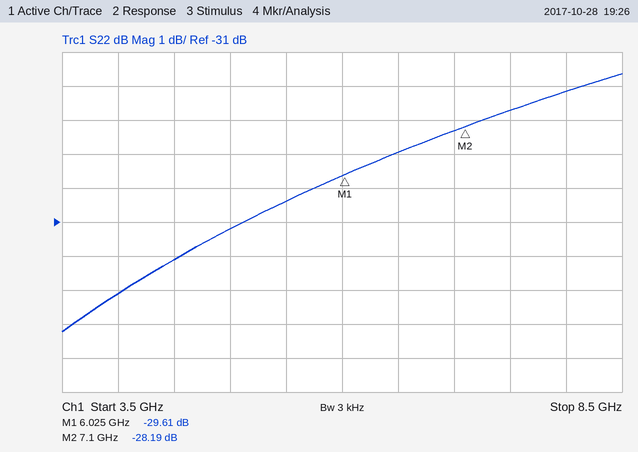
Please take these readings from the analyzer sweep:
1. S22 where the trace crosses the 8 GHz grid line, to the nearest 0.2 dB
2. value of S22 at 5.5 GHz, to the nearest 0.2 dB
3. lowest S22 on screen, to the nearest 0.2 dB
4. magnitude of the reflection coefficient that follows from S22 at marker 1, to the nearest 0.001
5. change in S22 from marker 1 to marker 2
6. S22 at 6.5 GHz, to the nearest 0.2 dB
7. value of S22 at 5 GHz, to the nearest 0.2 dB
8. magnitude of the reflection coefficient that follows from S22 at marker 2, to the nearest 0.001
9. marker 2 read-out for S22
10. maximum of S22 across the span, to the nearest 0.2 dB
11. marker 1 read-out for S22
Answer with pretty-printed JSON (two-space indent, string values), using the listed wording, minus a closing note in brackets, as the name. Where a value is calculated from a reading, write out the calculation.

{
  "S22 where the trace crosses the 8 GHz grid line, to the nearest 0.2 dB": "-27.2 dB",
  "value of S22 at 5.5 GHz, to the nearest 0.2 dB": "-30.4 dB",
  "lowest S22 on screen, to the nearest 0.2 dB": "-34.2 dB",
  "magnitude of the reflection coefficient that follows from S22 at marker 1, to the nearest 0.001": "10^(-29.61/20) ≈ 0.033",
  "change in S22 from marker 1 to marker 2": "-28.19 − (-29.61) = 1.42 dB",
  "S22 at 6.5 GHz, to the nearest 0.2 dB": "-29.0 dB",
  "value of S22 at 5 GHz, to the nearest 0.2 dB": "-31.2 dB",
  "magnitude of the reflection coefficient that follows from S22 at marker 2, to the nearest 0.001": "10^(-28.19/20) ≈ 0.039",
  "marker 2 read-out for S22": "-28.19 dB",
  "maximum of S22 across the span, to the nearest 0.2 dB": "-26.6 dB",
  "marker 1 read-out for S22": "-29.61 dB"
}
